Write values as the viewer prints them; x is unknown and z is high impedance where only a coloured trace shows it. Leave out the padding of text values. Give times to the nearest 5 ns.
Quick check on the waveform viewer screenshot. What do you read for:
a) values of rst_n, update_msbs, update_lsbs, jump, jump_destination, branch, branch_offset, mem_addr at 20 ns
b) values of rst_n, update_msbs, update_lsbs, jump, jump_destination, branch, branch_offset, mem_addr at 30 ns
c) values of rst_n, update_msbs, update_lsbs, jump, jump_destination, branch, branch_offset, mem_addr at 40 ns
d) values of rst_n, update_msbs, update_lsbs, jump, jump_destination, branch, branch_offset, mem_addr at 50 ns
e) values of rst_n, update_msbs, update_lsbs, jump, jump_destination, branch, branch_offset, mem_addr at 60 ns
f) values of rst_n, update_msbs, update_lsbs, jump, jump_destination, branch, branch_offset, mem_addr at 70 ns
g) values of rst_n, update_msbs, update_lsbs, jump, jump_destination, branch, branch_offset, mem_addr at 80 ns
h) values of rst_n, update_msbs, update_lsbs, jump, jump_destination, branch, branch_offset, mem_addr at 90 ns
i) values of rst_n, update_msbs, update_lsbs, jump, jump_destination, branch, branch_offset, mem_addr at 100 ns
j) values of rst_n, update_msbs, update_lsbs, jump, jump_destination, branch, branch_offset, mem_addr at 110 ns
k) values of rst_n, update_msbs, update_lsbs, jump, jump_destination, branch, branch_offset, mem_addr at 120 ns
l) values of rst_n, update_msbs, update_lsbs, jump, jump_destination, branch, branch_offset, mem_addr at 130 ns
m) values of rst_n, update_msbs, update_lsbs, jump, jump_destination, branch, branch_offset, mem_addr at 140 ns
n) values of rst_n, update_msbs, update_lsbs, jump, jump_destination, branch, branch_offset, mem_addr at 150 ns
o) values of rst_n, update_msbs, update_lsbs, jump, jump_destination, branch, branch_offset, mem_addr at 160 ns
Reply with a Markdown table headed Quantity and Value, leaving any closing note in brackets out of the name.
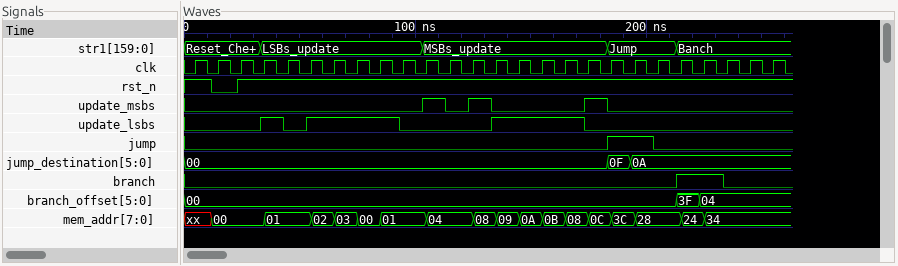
| Quantity | Value |
|---|---|
| values of rst_n, update_msbs, update_lsbs, jump, jump_destination, branch, branch_offset, mem_addr at 20 ns | rst_n=0, update_msbs=0, update_lsbs=0, jump=0, jump_destination=00, branch=0, branch_offset=00, mem_addr=00 |
| values of rst_n, update_msbs, update_lsbs, jump, jump_destination, branch, branch_offset, mem_addr at 30 ns | rst_n=1, update_msbs=0, update_lsbs=0, jump=0, jump_destination=00, branch=0, branch_offset=00, mem_addr=00 |
| values of rst_n, update_msbs, update_lsbs, jump, jump_destination, branch, branch_offset, mem_addr at 40 ns | rst_n=1, update_msbs=0, update_lsbs=1, jump=0, jump_destination=00, branch=0, branch_offset=00, mem_addr=01 |
| values of rst_n, update_msbs, update_lsbs, jump, jump_destination, branch, branch_offset, mem_addr at 50 ns | rst_n=1, update_msbs=0, update_lsbs=0, jump=0, jump_destination=00, branch=0, branch_offset=00, mem_addr=01 |
| values of rst_n, update_msbs, update_lsbs, jump, jump_destination, branch, branch_offset, mem_addr at 60 ns | rst_n=1, update_msbs=0, update_lsbs=1, jump=0, jump_destination=00, branch=0, branch_offset=00, mem_addr=02 |
| values of rst_n, update_msbs, update_lsbs, jump, jump_destination, branch, branch_offset, mem_addr at 70 ns | rst_n=1, update_msbs=0, update_lsbs=1, jump=0, jump_destination=00, branch=0, branch_offset=00, mem_addr=03 |
| values of rst_n, update_msbs, update_lsbs, jump, jump_destination, branch, branch_offset, mem_addr at 80 ns | rst_n=1, update_msbs=0, update_lsbs=1, jump=0, jump_destination=00, branch=0, branch_offset=00, mem_addr=00 |
| values of rst_n, update_msbs, update_lsbs, jump, jump_destination, branch, branch_offset, mem_addr at 90 ns | rst_n=1, update_msbs=0, update_lsbs=1, jump=0, jump_destination=00, branch=0, branch_offset=00, mem_addr=01 |
| values of rst_n, update_msbs, update_lsbs, jump, jump_destination, branch, branch_offset, mem_addr at 100 ns | rst_n=1, update_msbs=0, update_lsbs=0, jump=0, jump_destination=00, branch=0, branch_offset=00, mem_addr=01 |
| values of rst_n, update_msbs, update_lsbs, jump, jump_destination, branch, branch_offset, mem_addr at 110 ns | rst_n=1, update_msbs=1, update_lsbs=0, jump=0, jump_destination=00, branch=0, branch_offset=00, mem_addr=04 |
| values of rst_n, update_msbs, update_lsbs, jump, jump_destination, branch, branch_offset, mem_addr at 120 ns | rst_n=1, update_msbs=0, update_lsbs=0, jump=0, jump_destination=00, branch=0, branch_offset=00, mem_addr=04 |
| values of rst_n, update_msbs, update_lsbs, jump, jump_destination, branch, branch_offset, mem_addr at 130 ns | rst_n=1, update_msbs=1, update_lsbs=0, jump=0, jump_destination=00, branch=0, branch_offset=00, mem_addr=08 |
| values of rst_n, update_msbs, update_lsbs, jump, jump_destination, branch, branch_offset, mem_addr at 140 ns | rst_n=1, update_msbs=0, update_lsbs=1, jump=0, jump_destination=00, branch=0, branch_offset=00, mem_addr=09 |
| values of rst_n, update_msbs, update_lsbs, jump, jump_destination, branch, branch_offset, mem_addr at 150 ns | rst_n=1, update_msbs=0, update_lsbs=1, jump=0, jump_destination=00, branch=0, branch_offset=00, mem_addr=0A |
| values of rst_n, update_msbs, update_lsbs, jump, jump_destination, branch, branch_offset, mem_addr at 160 ns | rst_n=1, update_msbs=0, update_lsbs=1, jump=0, jump_destination=00, branch=0, branch_offset=00, mem_addr=0B |
